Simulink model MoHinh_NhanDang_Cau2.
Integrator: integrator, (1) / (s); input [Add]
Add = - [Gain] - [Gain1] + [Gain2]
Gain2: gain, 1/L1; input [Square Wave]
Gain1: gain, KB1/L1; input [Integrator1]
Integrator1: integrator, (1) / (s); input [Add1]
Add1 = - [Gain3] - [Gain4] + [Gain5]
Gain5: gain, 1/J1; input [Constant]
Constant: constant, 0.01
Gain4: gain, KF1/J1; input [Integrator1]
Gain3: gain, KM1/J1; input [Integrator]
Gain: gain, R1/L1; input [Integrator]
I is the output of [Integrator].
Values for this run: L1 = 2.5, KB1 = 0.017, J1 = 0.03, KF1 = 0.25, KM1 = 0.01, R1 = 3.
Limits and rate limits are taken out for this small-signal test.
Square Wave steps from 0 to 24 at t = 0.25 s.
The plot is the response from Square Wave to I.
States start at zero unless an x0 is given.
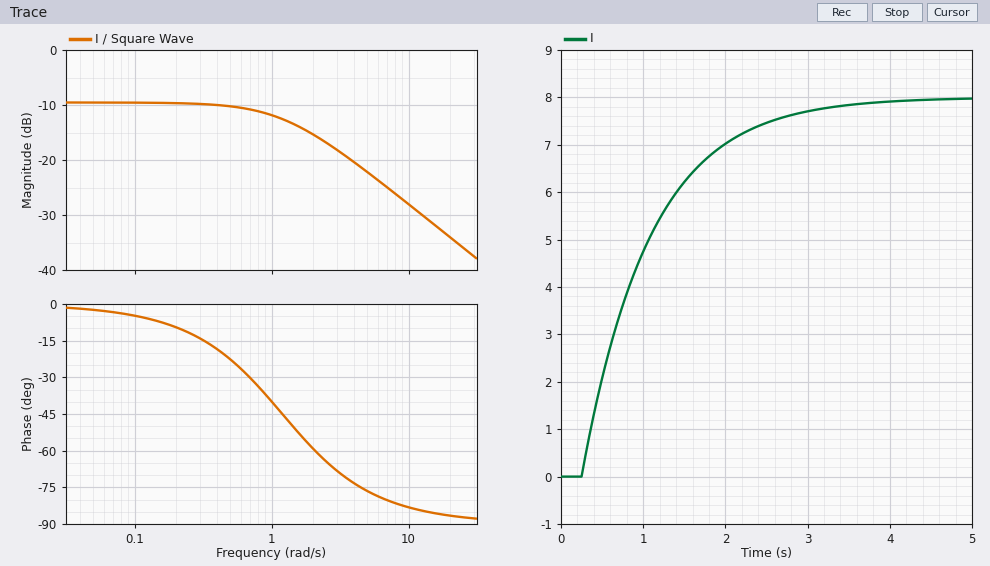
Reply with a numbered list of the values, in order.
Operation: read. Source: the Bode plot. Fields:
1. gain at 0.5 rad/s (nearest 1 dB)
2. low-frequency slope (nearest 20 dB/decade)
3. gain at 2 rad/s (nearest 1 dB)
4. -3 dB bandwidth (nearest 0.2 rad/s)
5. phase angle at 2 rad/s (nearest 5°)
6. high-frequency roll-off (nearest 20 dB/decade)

1. -10 dB
2. 0 dB/decade
3. -15 dB
4. 1.2 rad/s
5. -60°
6. -20 dB/decade
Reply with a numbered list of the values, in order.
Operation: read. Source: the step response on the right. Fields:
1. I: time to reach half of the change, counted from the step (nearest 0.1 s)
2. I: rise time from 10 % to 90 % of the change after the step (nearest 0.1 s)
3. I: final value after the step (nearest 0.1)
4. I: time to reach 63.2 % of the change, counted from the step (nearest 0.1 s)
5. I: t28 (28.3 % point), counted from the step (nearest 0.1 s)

1. 0.6 s
2. 1.8 s
3. 8.0
4. 0.8 s
5. 0.3 s
